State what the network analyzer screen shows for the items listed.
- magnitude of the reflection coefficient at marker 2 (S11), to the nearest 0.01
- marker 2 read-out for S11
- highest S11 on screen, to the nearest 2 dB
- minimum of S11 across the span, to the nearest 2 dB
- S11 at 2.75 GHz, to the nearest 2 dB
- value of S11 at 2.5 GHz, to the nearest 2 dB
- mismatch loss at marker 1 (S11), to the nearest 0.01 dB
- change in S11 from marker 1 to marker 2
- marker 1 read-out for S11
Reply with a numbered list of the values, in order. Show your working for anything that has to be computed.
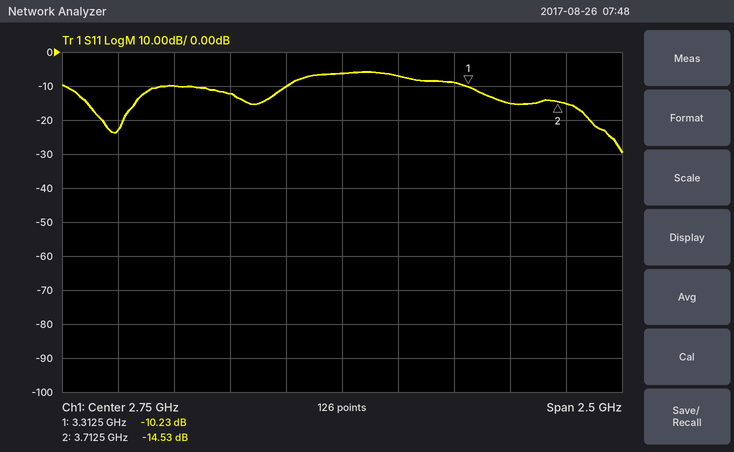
1. 10^(-14.53/20) ≈ 0.19
2. -14.53 dB
3. -6 dB
4. -30 dB
5. -6 dB
6. -10 dB
7. −10 log10(1 − 10^(-10.23/10)) ≈ 0.43 dB
8. -14.53 − (-10.23) = -4.30 dB
9. -10.23 dB
